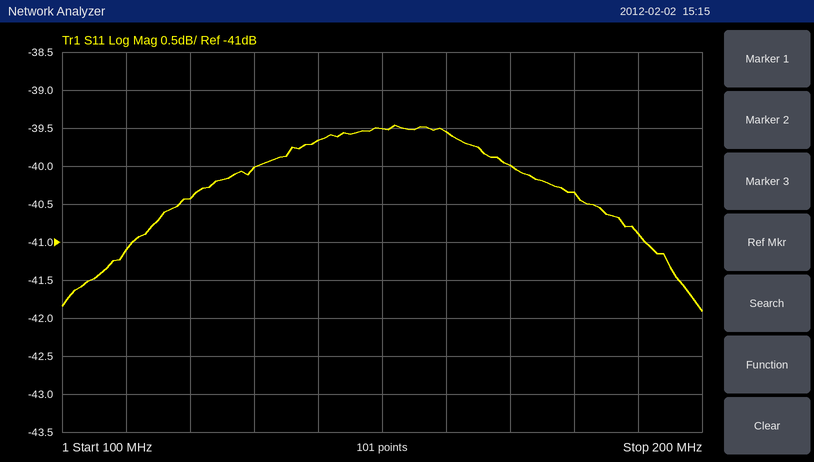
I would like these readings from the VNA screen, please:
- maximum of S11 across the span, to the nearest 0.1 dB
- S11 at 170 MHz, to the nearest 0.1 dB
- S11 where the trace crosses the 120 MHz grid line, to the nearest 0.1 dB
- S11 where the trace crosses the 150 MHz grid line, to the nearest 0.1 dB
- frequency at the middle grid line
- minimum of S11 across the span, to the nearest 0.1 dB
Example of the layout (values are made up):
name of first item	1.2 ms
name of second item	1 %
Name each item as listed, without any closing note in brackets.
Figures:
maximum of S11 across the span, to the nearest 0.1 dB	-39.5 dB
S11 at 170 MHz, to the nearest 0.1 dB	-40.0 dB
S11 where the trace crosses the 120 MHz grid line, to the nearest 0.1 dB	-40.4 dB
S11 where the trace crosses the 150 MHz grid line, to the nearest 0.1 dB	-39.5 dB
frequency at the middle grid line	150 MHz
minimum of S11 across the span, to the nearest 0.1 dB	-41.9 dB
